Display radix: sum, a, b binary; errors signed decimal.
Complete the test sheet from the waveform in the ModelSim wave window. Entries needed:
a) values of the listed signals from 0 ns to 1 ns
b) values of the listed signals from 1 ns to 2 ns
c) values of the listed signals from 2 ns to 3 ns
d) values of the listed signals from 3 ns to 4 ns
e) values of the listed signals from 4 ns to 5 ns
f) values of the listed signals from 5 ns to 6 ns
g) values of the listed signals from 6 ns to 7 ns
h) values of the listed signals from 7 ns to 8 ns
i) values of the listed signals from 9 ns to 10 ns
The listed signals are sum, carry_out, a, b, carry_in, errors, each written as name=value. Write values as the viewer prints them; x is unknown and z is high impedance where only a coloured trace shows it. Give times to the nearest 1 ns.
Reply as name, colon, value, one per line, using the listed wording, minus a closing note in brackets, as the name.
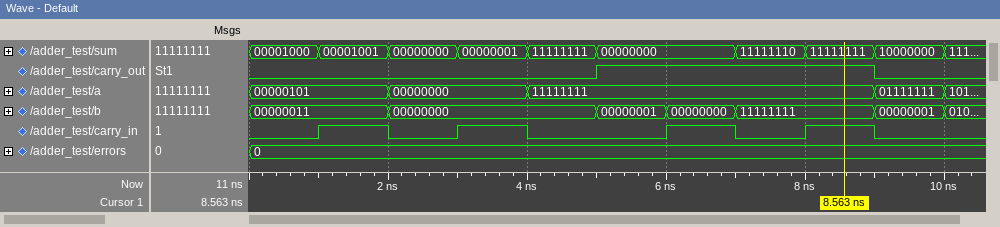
values of the listed signals from 0 ns to 1 ns: sum=00001000, carry_out=0, a=00000101, b=00000011, carry_in=0, errors=0
values of the listed signals from 1 ns to 2 ns: sum=00001001, carry_out=0, a=00000101, b=00000011, carry_in=1, errors=0
values of the listed signals from 2 ns to 3 ns: sum=00000000, carry_out=0, a=00000000, b=00000000, carry_in=0, errors=0
values of the listed signals from 3 ns to 4 ns: sum=00000001, carry_out=0, a=00000000, b=00000000, carry_in=1, errors=0
values of the listed signals from 4 ns to 5 ns: sum=11111111, carry_out=0, a=11111111, b=00000000, carry_in=0, errors=0
values of the listed signals from 5 ns to 6 ns: sum=00000000, carry_out=1, a=11111111, b=00000001, carry_in=0, errors=0
values of the listed signals from 6 ns to 7 ns: sum=00000000, carry_out=1, a=11111111, b=00000000, carry_in=1, errors=0
values of the listed signals from 7 ns to 8 ns: sum=11111110, carry_out=1, a=11111111, b=11111111, carry_in=0, errors=0
values of the listed signals from 9 ns to 10 ns: sum=10000000, carry_out=0, a=01111111, b=00000001, carry_in=0, errors=0
